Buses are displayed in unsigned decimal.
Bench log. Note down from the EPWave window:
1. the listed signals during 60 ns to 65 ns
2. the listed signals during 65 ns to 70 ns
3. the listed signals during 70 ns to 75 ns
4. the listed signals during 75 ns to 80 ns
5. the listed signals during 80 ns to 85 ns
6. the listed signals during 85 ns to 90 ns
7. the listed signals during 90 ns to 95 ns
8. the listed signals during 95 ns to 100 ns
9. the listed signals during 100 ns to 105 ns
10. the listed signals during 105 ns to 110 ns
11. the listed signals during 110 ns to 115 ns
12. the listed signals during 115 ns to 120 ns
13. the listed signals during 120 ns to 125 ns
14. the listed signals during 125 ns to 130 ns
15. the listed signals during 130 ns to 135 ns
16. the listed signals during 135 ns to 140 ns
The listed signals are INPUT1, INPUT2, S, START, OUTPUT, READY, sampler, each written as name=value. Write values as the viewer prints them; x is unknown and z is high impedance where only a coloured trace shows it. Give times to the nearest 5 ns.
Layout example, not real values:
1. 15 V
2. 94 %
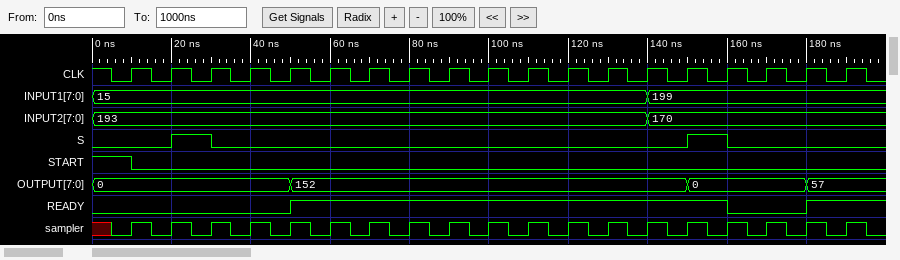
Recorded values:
1. INPUT1=15, INPUT2=193, S=0, START=0, OUTPUT=152, READY=1, sampler=1
2. INPUT1=15, INPUT2=193, S=0, START=0, OUTPUT=152, READY=1, sampler=0
3. INPUT1=15, INPUT2=193, S=0, START=0, OUTPUT=152, READY=1, sampler=1
4. INPUT1=15, INPUT2=193, S=0, START=0, OUTPUT=152, READY=1, sampler=0
5. INPUT1=15, INPUT2=193, S=0, START=0, OUTPUT=152, READY=1, sampler=1
6. INPUT1=15, INPUT2=193, S=0, START=0, OUTPUT=152, READY=1, sampler=0
7. INPUT1=15, INPUT2=193, S=0, START=0, OUTPUT=152, READY=1, sampler=1
8. INPUT1=15, INPUT2=193, S=0, START=0, OUTPUT=152, READY=1, sampler=0
9. INPUT1=15, INPUT2=193, S=0, START=0, OUTPUT=152, READY=1, sampler=1
10. INPUT1=15, INPUT2=193, S=0, START=0, OUTPUT=152, READY=1, sampler=0
11. INPUT1=15, INPUT2=193, S=0, START=0, OUTPUT=152, READY=1, sampler=1
12. INPUT1=15, INPUT2=193, S=0, START=0, OUTPUT=152, READY=1, sampler=0
13. INPUT1=15, INPUT2=193, S=0, START=0, OUTPUT=152, READY=1, sampler=1
14. INPUT1=15, INPUT2=193, S=0, START=0, OUTPUT=152, READY=1, sampler=0
15. INPUT1=15, INPUT2=193, S=0, START=0, OUTPUT=152, READY=1, sampler=1
16. INPUT1=15, INPUT2=193, S=0, START=0, OUTPUT=152, READY=1, sampler=0
